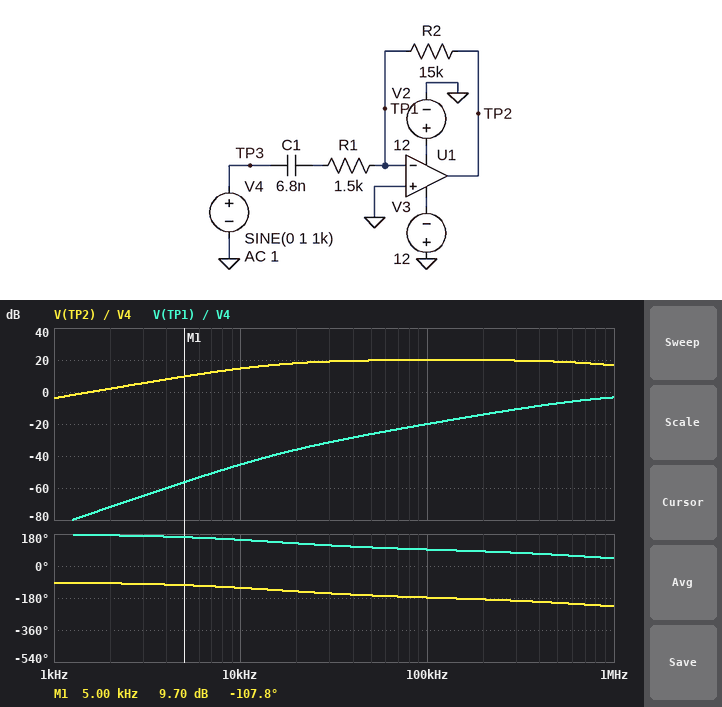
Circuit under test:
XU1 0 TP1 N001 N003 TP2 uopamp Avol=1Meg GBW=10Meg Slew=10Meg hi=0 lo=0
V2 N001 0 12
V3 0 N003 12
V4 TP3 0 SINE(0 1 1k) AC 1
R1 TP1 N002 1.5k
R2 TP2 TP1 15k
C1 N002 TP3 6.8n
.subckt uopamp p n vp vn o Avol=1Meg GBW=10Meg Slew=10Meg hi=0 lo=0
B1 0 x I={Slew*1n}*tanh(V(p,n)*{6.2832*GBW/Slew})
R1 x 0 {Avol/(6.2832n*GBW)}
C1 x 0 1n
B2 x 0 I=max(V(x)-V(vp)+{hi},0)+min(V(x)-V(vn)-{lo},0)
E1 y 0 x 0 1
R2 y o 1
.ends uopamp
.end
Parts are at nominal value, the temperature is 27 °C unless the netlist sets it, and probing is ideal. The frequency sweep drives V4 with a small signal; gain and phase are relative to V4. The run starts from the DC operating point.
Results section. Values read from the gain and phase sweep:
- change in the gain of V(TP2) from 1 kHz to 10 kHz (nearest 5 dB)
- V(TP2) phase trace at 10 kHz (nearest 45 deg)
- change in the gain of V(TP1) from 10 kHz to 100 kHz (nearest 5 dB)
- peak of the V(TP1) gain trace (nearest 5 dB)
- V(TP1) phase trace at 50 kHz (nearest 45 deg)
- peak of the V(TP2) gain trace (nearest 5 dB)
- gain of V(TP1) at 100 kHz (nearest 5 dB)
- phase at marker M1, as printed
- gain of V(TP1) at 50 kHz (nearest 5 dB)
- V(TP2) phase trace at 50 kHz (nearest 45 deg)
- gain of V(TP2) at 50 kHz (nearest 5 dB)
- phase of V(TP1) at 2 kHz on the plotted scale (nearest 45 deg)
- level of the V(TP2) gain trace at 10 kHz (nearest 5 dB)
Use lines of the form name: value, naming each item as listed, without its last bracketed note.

change in the gain of V(TP2) from 1 kHz to 10 kHz: 20 dB
V(TP2) phase trace at 10 kHz: -135 deg
change in the gain of V(TP1) from 10 kHz to 100 kHz: 25 dB
peak of the V(TP1) gain trace: -5 dB
V(TP1) phase trace at 50 kHz: 90 deg
peak of the V(TP2) gain trace: 20 dB
gain of V(TP1) at 100 kHz: -20 dB
phase at marker M1, as printed: -107.8 deg
gain of V(TP1) at 50 kHz: -25 dB
V(TP2) phase trace at 50 kHz: -180 deg
gain of V(TP2) at 50 kHz: 20 dB
phase of V(TP1) at 2 kHz on the plotted scale: 180 deg
level of the V(TP2) gain trace at 10 kHz: 15 dB
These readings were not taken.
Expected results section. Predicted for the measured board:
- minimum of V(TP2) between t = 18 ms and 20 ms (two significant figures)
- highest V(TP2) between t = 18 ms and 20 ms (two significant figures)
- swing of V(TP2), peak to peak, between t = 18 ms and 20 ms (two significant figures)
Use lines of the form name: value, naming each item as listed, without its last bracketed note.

minimum of V(TP2) between t = 18 ms and 20 ms: -640 mV
highest V(TP2) between t = 18 ms and 20 ms: 640 mV
swing of V(TP2), peak to peak, between t = 18 ms and 20 ms: 1.3 V
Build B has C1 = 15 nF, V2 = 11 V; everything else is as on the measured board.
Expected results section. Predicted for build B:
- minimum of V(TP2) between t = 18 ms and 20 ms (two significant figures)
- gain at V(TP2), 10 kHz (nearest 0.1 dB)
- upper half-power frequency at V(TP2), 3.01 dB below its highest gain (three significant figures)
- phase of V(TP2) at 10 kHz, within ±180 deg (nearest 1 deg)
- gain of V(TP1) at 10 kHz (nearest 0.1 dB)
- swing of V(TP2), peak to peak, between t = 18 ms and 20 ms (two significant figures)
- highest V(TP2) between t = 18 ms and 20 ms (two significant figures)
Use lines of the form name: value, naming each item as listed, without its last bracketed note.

minimum of V(TP2) between t = 18 ms and 20 ms: -1.4 V
gain at V(TP2), 10 kHz: 18.3 dB
upper half-power frequency at V(TP2), 3.01 dB below its highest gain: 917 kHz
phase of V(TP2) at 10 kHz, within ±180 deg: -145 deg
gain of V(TP1) at 10 kHz: -41.7 dB
swing of V(TP2), peak to peak, between t = 18 ms and 20 ms: 2.8 V
highest V(TP2) between t = 18 ms and 20 ms: 1.4 V
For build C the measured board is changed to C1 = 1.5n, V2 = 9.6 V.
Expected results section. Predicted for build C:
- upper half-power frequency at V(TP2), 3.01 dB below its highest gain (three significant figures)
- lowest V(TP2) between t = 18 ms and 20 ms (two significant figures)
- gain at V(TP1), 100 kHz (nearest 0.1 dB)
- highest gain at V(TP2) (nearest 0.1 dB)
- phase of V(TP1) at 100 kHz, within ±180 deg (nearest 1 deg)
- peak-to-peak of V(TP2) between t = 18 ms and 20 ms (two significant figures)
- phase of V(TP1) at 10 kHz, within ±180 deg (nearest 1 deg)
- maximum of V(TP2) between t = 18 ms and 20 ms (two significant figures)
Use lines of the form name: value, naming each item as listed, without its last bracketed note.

upper half-power frequency at V(TP2), 3.01 dB below its highest gain: 981 kHz
lowest V(TP2) between t = 18 ms and 20 ms: -140 mV
gain at V(TP1), 100 kHz: -21.4 dB
highest gain at V(TP2): 19.9 dB
phase of V(TP1) at 100 kHz, within ±180 deg: 121 deg
peak-to-peak of V(TP2) between t = 18 ms and 20 ms: 280 mV
phase of V(TP1) at 10 kHz, within ±180 deg: 172 deg
maximum of V(TP2) between t = 18 ms and 20 ms: 140 mV
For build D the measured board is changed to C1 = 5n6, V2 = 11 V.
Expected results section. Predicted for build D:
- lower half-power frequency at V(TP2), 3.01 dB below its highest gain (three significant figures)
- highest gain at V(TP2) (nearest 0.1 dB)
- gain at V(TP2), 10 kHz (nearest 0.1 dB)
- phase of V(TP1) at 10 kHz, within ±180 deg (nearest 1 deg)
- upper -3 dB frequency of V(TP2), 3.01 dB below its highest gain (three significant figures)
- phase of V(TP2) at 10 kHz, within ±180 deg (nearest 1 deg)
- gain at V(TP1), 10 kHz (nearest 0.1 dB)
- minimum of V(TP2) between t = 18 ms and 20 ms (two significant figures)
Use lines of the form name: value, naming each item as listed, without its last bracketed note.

lower half-power frequency at V(TP2), 3.01 dB below its highest gain: 18.5 kHz
highest gain at V(TP2): 20.0 dB
gain at V(TP2), 10 kHz: 13.4 dB
phase of V(TP1) at 10 kHz, within ±180 deg: 152 deg
upper -3 dB frequency of V(TP2), 3.01 dB below its highest gain: 929 kHz
phase of V(TP2) at 10 kHz, within ±180 deg: -118 deg
gain at V(TP1), 10 kHz: -46.6 dB
minimum of V(TP2) between t = 18 ms and 20 ms: -530 mV
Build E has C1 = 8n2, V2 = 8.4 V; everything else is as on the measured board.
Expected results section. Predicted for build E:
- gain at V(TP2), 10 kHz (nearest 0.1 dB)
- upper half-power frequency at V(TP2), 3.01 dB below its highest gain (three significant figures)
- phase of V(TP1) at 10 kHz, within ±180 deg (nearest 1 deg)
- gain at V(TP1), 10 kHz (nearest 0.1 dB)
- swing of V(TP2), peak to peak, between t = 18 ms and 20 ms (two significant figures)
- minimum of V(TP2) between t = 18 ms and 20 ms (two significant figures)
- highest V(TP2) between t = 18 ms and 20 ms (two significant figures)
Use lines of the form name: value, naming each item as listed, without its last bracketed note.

gain at V(TP2), 10 kHz: 15.8 dB
upper half-power frequency at V(TP2), 3.01 dB below its highest gain: 923 kHz
phase of V(TP1) at 10 kHz, within ±180 deg: 142 deg
gain at V(TP1), 10 kHz: -44.2 dB
swing of V(TP2), peak to peak, between t = 18 ms and 20 ms: 1.5 V
minimum of V(TP2) between t = 18 ms and 20 ms: -770 mV
highest V(TP2) between t = 18 ms and 20 ms: 770 mV
